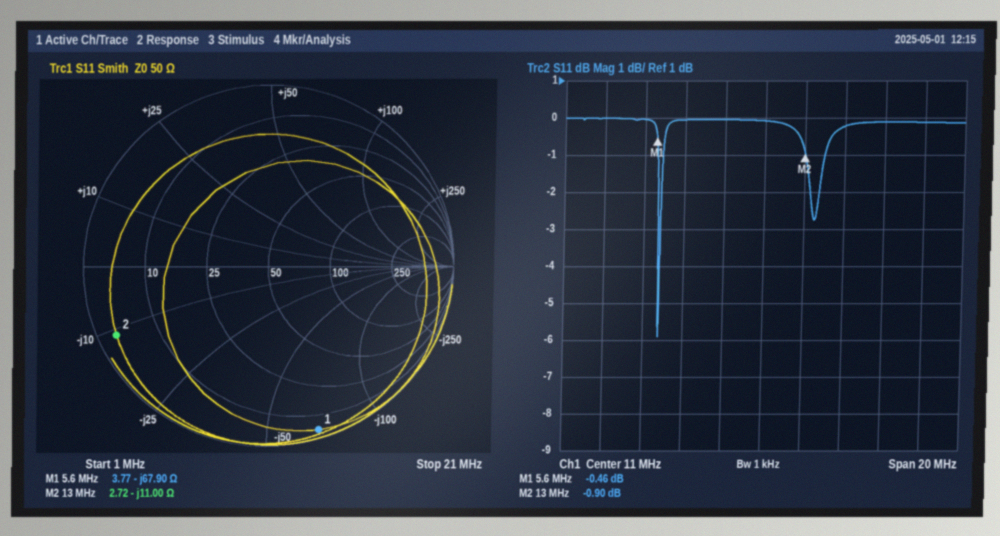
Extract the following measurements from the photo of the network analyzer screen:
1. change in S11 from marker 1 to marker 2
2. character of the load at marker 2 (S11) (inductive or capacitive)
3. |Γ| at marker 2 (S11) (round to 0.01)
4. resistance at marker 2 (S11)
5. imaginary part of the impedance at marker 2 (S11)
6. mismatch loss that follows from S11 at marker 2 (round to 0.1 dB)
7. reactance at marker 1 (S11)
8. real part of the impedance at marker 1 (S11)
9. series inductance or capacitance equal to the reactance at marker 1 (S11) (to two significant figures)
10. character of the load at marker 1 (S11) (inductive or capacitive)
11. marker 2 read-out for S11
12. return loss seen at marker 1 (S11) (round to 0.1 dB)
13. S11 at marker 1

-0.44 dB
capacitive
0.90
2.72 Ω
-11.00 Ω
7.3 dB
-67.90 Ω
3.77 Ω
420 pF
capacitive
-0.90 dB
0.5 dB
-0.46 dB
